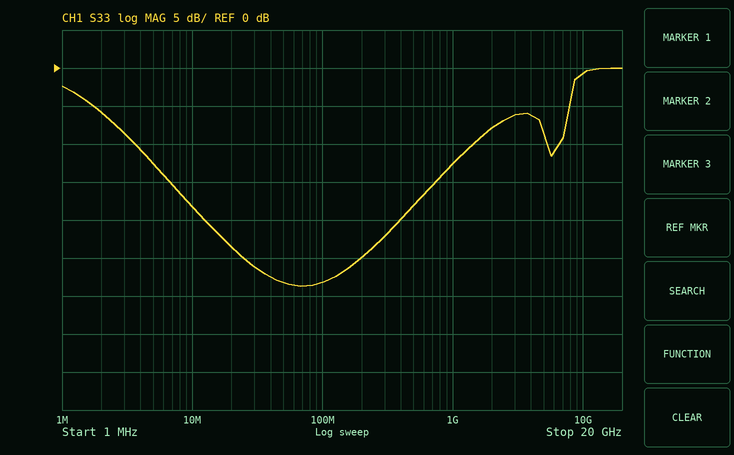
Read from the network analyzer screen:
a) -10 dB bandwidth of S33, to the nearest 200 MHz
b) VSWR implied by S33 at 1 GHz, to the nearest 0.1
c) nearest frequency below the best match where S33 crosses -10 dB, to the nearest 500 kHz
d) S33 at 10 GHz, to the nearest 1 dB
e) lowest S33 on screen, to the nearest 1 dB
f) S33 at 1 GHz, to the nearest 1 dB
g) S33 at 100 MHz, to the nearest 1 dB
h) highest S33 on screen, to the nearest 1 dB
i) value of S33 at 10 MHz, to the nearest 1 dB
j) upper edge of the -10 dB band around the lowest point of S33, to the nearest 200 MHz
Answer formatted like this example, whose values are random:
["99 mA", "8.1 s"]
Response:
["1.4 GHz", "1.6", "3.5 MHz", "-1 dB", "-29 dB", "-13 dB", "-28 dB", "0 dB", "-18 dB", "1.4 GHz"]
